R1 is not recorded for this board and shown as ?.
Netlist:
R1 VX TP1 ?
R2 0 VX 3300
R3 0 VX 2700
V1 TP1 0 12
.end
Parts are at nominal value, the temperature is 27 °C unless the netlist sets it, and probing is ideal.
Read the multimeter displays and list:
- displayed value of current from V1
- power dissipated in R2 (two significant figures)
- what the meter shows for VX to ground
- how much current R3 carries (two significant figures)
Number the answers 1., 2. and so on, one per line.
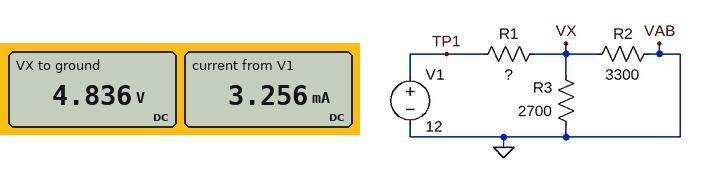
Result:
1. 3.256 mA
2. 7.1 mW
3. 4.836 V
4. 1.8 mA
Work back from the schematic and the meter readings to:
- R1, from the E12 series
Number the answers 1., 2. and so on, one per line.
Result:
1. 2.2 kΩ
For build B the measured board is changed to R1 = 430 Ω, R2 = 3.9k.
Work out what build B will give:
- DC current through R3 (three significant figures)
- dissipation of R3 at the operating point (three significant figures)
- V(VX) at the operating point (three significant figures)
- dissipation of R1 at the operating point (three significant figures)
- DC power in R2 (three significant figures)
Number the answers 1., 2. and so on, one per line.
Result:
1. 3.50 mA
2. 33.1 mW
3. 9.45 V
4. 15.1 mW
5. 22.9 mW
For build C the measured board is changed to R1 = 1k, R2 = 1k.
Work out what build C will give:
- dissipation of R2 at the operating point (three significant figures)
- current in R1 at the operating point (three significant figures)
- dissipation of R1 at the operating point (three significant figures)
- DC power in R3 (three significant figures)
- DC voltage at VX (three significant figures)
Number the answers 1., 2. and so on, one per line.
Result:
1. 25.6 mW
2. 6.94 mA
3. 48.1 mW
4. 9.49 mW
5. 5.06 V
